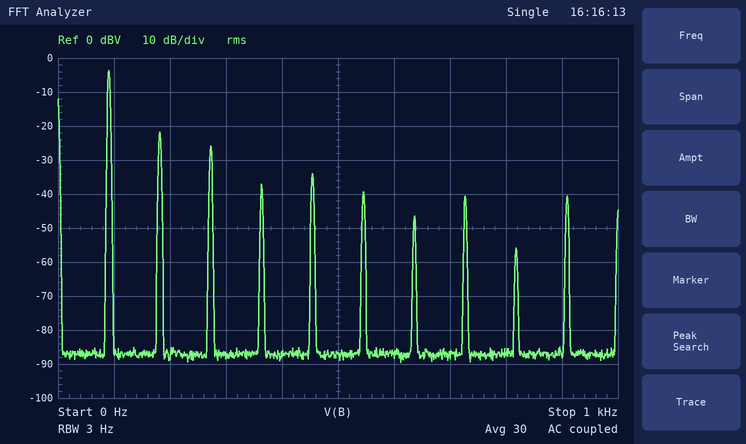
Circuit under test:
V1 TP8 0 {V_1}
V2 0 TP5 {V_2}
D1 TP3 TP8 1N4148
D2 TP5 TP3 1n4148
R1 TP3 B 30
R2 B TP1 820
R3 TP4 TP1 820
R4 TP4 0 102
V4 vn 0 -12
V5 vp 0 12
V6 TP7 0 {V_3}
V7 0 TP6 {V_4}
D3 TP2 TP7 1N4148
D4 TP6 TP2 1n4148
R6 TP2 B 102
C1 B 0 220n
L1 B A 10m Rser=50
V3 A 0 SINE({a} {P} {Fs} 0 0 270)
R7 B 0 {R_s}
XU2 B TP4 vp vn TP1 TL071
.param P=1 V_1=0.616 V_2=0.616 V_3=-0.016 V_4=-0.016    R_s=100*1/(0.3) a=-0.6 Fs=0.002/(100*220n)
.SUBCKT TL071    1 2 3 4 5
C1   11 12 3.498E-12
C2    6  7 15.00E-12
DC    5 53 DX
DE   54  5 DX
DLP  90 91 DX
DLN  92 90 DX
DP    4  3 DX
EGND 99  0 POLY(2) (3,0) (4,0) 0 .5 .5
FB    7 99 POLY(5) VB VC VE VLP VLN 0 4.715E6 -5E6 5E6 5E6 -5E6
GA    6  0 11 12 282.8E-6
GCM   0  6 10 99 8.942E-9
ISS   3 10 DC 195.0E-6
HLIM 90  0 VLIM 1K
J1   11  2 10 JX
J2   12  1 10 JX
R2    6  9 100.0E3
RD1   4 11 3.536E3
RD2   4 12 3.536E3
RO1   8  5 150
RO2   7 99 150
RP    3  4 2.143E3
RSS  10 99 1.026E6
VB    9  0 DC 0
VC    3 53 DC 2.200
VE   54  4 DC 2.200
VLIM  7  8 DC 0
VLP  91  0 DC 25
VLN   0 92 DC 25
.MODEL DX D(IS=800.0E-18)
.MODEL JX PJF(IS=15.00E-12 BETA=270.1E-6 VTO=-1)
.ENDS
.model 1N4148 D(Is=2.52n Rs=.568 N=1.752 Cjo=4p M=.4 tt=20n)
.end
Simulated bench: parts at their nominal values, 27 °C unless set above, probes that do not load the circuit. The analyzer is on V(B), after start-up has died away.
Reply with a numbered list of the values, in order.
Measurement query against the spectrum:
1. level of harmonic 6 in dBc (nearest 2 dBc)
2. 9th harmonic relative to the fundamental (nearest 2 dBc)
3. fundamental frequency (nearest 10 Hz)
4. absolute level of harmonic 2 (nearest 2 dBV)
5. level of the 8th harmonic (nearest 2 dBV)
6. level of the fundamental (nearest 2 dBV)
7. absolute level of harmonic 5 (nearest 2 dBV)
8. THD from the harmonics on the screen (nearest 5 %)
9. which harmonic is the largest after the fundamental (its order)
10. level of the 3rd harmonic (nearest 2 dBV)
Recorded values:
1. -36 dBc
2. -52 dBc
3. 90 Hz
4. -22 dBV
5. -40 dBV
6. -4 dBV
7. -34 dBV
8. 15 %
9. 2
10. -26 dBV
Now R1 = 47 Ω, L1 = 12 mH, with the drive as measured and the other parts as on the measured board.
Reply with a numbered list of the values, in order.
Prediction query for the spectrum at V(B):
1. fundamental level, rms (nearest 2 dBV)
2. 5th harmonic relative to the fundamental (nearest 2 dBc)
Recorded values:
1. -4 dBV
2. -28 dBc
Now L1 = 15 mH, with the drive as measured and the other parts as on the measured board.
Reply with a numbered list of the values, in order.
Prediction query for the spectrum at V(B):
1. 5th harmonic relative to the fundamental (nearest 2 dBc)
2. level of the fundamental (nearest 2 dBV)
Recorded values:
1. -26 dBc
2. -4 dBV
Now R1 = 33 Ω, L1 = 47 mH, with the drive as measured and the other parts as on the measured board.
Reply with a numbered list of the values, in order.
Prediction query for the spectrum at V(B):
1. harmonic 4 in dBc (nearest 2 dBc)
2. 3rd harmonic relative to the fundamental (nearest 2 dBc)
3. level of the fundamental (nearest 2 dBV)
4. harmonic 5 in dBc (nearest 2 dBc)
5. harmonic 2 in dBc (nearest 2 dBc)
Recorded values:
1. -26 dBc
2. -18 dBc
3. -4 dBV
4. -20 dBc
5. -16 dBc
